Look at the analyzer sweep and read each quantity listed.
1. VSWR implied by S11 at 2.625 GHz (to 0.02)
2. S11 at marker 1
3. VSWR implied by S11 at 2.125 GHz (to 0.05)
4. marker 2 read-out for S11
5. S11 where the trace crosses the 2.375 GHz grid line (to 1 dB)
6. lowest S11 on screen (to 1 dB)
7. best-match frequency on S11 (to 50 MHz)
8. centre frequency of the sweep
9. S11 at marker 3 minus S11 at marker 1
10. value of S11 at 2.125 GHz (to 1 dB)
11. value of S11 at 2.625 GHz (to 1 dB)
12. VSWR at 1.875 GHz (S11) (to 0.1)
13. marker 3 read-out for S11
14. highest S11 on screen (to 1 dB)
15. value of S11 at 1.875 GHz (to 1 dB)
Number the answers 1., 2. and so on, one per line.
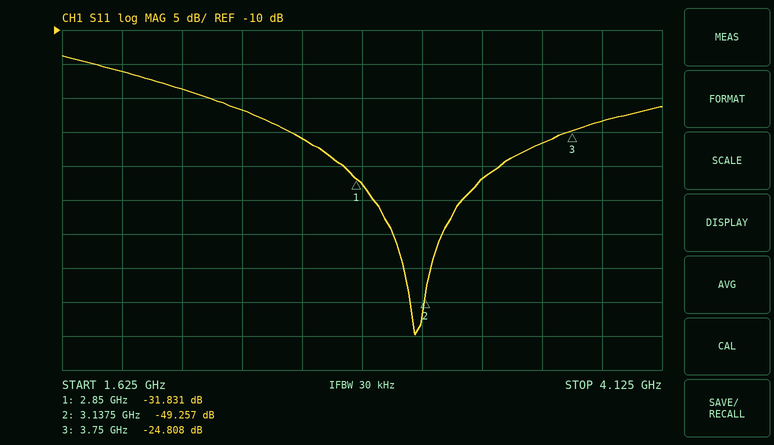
1. 1.10
2. -31.831 dB
3. 1.25
4. -49.257 dB
5. -22 dB
6. -55 dB
7. 3.10 GHz
8. 2.875 GHz
9. 7.023 dB
10. -19 dB
11. -26 dB
12. 1.4
13. -24.808 dB
14. -14 dB
15. -16 dB
